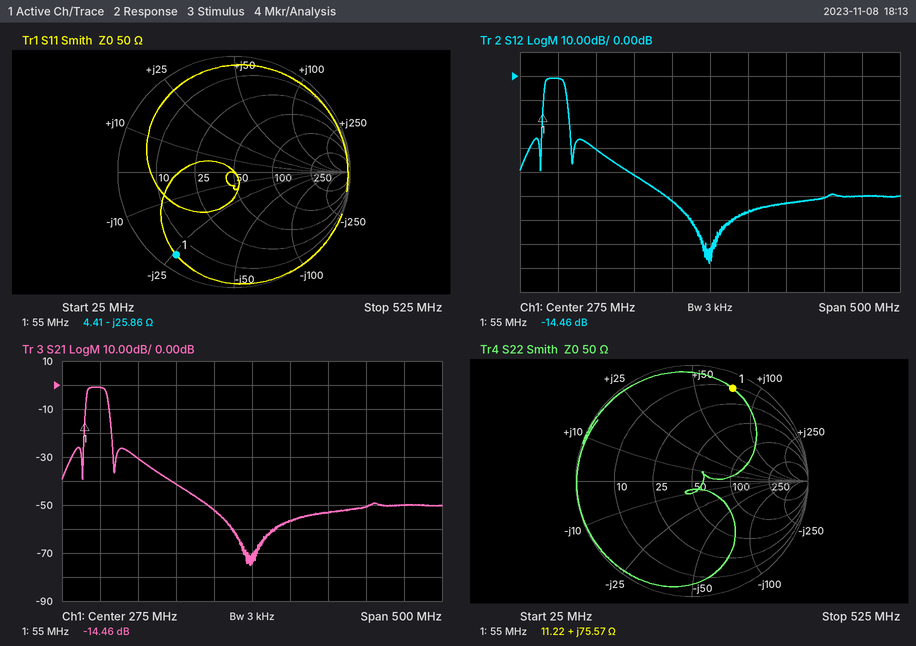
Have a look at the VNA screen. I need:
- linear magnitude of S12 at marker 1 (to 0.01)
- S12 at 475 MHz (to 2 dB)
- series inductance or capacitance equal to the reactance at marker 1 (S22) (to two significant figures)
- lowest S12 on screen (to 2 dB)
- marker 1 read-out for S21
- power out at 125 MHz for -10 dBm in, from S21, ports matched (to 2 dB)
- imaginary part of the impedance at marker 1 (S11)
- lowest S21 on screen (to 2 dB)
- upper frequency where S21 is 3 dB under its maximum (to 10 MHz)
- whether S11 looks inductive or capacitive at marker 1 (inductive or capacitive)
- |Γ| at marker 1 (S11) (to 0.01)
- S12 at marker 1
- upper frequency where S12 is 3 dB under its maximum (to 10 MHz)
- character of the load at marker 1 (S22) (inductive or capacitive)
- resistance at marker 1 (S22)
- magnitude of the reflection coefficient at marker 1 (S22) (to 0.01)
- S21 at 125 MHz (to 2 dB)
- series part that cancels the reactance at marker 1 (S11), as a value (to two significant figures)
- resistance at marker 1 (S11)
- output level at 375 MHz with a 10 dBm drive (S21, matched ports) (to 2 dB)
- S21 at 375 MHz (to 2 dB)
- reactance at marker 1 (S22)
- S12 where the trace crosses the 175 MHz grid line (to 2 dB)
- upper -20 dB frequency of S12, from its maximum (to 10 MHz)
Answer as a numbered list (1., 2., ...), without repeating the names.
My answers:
1. 0.19
2. -50 dB
3. 220 nH
4. -78 dB
5. -14.46 dB
6. -40 dBm
7. -25.86 Ω
8. -76 dB
9. 80 MHz
10. capacitive
11. 0.87
12. -14.46 dB
13. 80 MHz
14. inductive
15. 11.22 Ω
16. 0.87
17. -30 dB
18. 75 nH
19. 4.41 Ω
20. -44 dBm
21. -54 dB
22. +75.57 Ω
23. -42 dB
24. 90 MHz
